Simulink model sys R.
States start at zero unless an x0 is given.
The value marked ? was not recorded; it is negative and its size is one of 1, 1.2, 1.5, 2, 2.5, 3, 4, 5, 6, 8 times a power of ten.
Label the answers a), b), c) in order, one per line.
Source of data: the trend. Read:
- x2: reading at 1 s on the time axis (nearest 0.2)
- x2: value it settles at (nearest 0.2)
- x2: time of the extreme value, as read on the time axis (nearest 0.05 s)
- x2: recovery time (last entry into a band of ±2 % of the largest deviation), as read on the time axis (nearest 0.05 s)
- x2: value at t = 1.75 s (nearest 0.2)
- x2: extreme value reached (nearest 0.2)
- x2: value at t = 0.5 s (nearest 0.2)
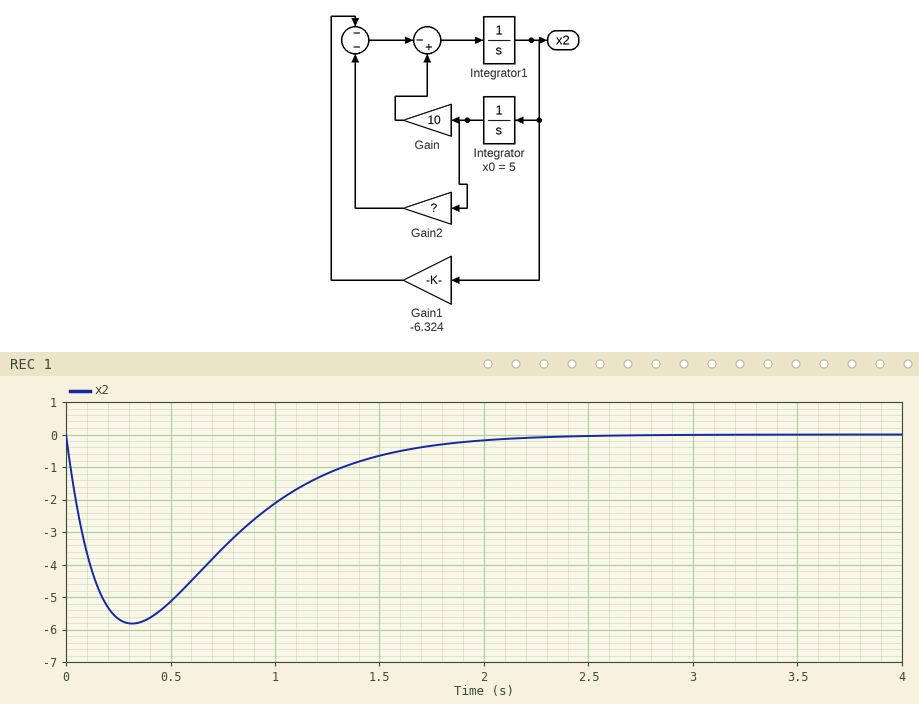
a) -2.2
b) 0.0
c) 0.30 s
d) 2.15 s
e) -0.4
f) -5.8
g) -5.2
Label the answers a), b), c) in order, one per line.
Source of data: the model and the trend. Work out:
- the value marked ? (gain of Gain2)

a) -20
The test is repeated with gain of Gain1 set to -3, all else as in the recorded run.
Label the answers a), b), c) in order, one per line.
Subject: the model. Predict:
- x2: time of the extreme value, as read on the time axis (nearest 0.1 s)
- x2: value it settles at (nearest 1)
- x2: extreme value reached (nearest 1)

a) 0.4 s
b) 0
c) -9
